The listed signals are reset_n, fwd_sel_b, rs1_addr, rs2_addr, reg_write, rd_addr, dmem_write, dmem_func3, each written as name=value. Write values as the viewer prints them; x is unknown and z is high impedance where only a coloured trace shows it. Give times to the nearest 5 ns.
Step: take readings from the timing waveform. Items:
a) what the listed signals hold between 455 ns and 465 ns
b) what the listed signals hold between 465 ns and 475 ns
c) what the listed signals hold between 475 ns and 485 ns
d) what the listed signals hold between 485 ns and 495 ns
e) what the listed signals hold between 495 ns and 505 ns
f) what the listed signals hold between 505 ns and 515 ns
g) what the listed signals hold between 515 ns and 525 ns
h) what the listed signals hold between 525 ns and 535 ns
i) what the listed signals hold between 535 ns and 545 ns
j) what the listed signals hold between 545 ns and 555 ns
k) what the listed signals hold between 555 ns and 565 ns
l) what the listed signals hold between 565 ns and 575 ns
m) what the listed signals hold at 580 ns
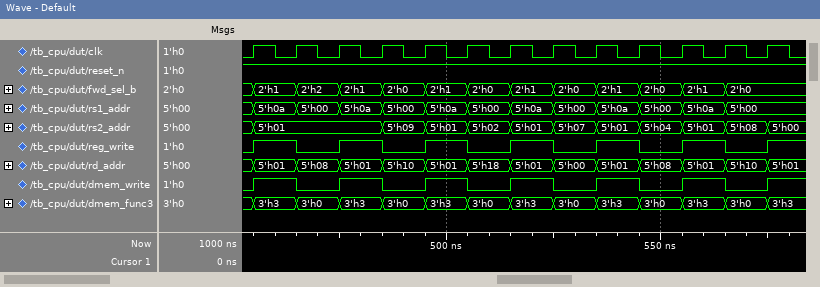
reset_n=1, fwd_sel_b=2'h1, rs1_addr=5'h0a, rs2_addr=5'h01, reg_write=1, rd_addr=5'h01, dmem_write=1, dmem_func3=3'h3
reset_n=1, fwd_sel_b=2'h2, rs1_addr=5'h00, rs2_addr=5'h01, reg_write=0, rd_addr=5'h08, dmem_write=0, dmem_func3=3'h0
reset_n=1, fwd_sel_b=2'h1, rs1_addr=5'h0a, rs2_addr=5'h01, reg_write=1, rd_addr=5'h01, dmem_write=1, dmem_func3=3'h3
reset_n=1, fwd_sel_b=2'h0, rs1_addr=5'h00, rs2_addr=5'h09, reg_write=0, rd_addr=5'h10, dmem_write=0, dmem_func3=3'h0
reset_n=1, fwd_sel_b=2'h1, rs1_addr=5'h0a, rs2_addr=5'h01, reg_write=1, rd_addr=5'h01, dmem_write=1, dmem_func3=3'h3
reset_n=1, fwd_sel_b=2'h0, rs1_addr=5'h00, rs2_addr=5'h02, reg_write=0, rd_addr=5'h18, dmem_write=0, dmem_func3=3'h0
reset_n=1, fwd_sel_b=2'h1, rs1_addr=5'h0a, rs2_addr=5'h01, reg_write=1, rd_addr=5'h01, dmem_write=1, dmem_func3=3'h3
reset_n=1, fwd_sel_b=2'h0, rs1_addr=5'h00, rs2_addr=5'h07, reg_write=0, rd_addr=5'h00, dmem_write=0, dmem_func3=3'h0
reset_n=1, fwd_sel_b=2'h1, rs1_addr=5'h0a, rs2_addr=5'h01, reg_write=1, rd_addr=5'h01, dmem_write=1, dmem_func3=3'h3
reset_n=1, fwd_sel_b=2'h0, rs1_addr=5'h00, rs2_addr=5'h04, reg_write=0, rd_addr=5'h08, dmem_write=0, dmem_func3=3'h0
reset_n=1, fwd_sel_b=2'h1, rs1_addr=5'h0a, rs2_addr=5'h01, reg_write=1, rd_addr=5'h01, dmem_write=1, dmem_func3=3'h3
reset_n=1, fwd_sel_b=2'h0, rs1_addr=5'h00, rs2_addr=5'h08, reg_write=0, rd_addr=5'h10, dmem_write=0, dmem_func3=3'h0
reset_n=1, fwd_sel_b=2'h0, rs1_addr=5'h00, rs2_addr=5'h00, reg_write=1, rd_addr=5'h01, dmem_write=1, dmem_func3=3'h3
